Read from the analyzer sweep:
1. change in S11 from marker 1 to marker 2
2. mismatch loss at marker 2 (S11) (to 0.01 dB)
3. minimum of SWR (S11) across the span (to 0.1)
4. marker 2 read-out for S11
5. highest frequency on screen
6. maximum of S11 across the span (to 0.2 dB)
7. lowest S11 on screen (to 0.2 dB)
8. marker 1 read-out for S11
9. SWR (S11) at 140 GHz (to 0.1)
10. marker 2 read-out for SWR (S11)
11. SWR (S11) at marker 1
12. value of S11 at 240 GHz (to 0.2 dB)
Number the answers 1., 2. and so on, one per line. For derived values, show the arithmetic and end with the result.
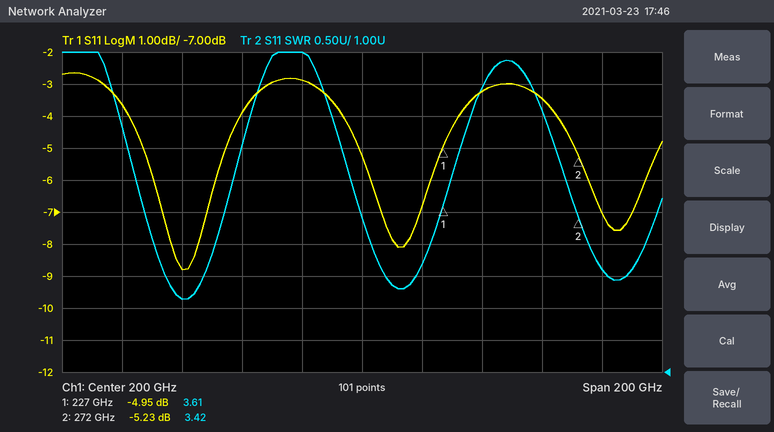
1. -5.23 − (-4.95) = -0.28 dB
2. −10 log10(1 − 10^(-5.23/10)) ≈ 1.55 dB
3. 2.1
4. -5.23 dB
5. 300 GHz
6. -2.6 dB
7. -8.8 dB
8. -4.95 dB
9. 2.1
10. 3.42
11. 3.61
12. -3.2 dB
